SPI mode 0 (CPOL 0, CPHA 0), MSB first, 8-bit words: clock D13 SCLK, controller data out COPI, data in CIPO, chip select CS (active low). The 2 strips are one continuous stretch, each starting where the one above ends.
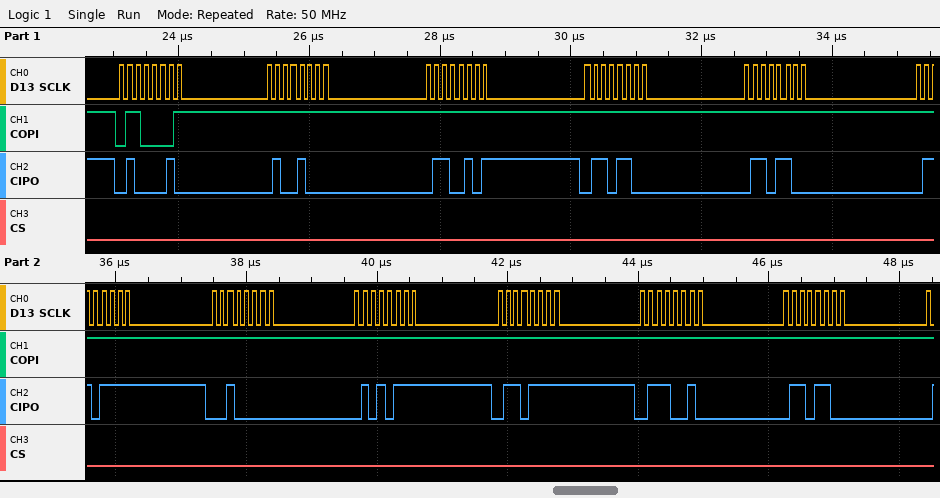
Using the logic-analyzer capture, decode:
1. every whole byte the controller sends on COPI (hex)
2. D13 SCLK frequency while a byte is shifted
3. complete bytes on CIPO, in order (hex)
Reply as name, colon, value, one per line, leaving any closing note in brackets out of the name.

every whole byte the controller sends on COPI: 61 FF FF FF FF FF FF FF FF FF FF
D13 SCLK frequency while a byte is shifted: 8 MHz
complete bytes on CIPO, in order: 42 48 65 6C 6C 6F 20 57 6F 72 6C
